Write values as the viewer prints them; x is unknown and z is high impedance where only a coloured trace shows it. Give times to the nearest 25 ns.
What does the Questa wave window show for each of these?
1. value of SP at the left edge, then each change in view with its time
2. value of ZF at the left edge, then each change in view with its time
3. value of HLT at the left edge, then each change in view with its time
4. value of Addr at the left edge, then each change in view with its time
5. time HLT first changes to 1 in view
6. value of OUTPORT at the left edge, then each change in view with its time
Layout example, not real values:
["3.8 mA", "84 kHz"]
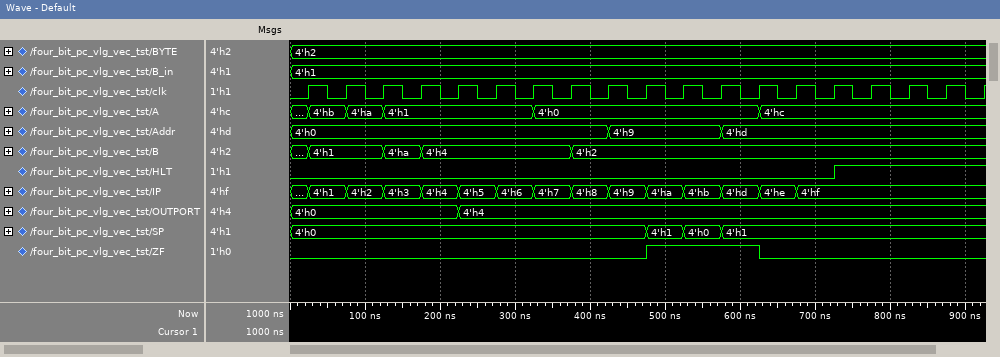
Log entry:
["4'h0, 4'h1 at 475 ns, 4'h0 at 525 ns, 4'h1 at 575 ns", "0, 1 at 475 ns, 0 at 625 ns", "0, 1 at 725 ns", "4'h0, 4'h9 at 425 ns, 4'hd at 575 ns", "725 ns", "4'h0, 4'h4 at 225 ns"]
